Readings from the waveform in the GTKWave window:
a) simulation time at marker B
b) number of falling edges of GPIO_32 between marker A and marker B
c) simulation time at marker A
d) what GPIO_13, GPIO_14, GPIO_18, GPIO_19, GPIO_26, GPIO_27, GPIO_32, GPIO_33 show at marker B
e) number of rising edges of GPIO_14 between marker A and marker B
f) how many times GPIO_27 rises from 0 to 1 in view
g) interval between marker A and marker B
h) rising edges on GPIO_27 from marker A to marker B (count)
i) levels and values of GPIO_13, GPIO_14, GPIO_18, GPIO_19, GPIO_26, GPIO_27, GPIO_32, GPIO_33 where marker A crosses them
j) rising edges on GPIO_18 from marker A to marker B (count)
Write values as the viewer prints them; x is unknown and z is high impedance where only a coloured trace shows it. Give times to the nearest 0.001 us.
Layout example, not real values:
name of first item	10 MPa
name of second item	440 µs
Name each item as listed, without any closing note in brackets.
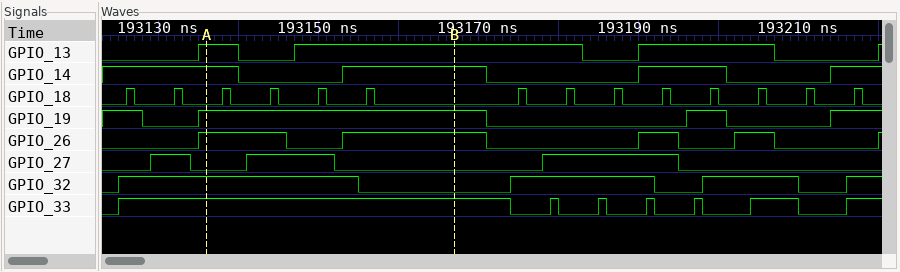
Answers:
simulation time at marker B	193.167 us
number of falling edges of GPIO_32 between marker A and marker B	1
simulation time at marker A	193.136 us
what GPIO_13, GPIO_14, GPIO_18, GPIO_19, GPIO_26, GPIO_27, GPIO_32, GPIO_33 show at marker B	GPIO_13=1, GPIO_14=1, GPIO_18=0, GPIO_19=1, GPIO_26=1, GPIO_27=0, GPIO_32=0, GPIO_33=1
number of rising edges of GPIO_14 between marker A and marker B	1
how many times GPIO_27 rises from 0 to 1 in view	3
interval between marker A and marker B	0.031 us
rising edges on GPIO_27 from marker A to marker B	1
levels and values of GPIO_13, GPIO_14, GPIO_18, GPIO_19, GPIO_26, GPIO_27, GPIO_32, GPIO_33 where marker A crosses them	GPIO_13=1, GPIO_14=1, GPIO_18=0, GPIO_19=1, GPIO_26=1, GPIO_27=0, GPIO_32=1, GPIO_33=1
rising edges on GPIO_18 from marker A to marker B	4
